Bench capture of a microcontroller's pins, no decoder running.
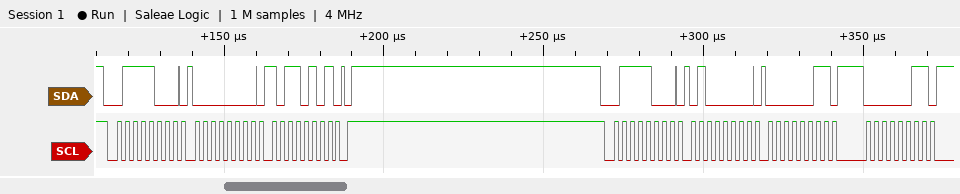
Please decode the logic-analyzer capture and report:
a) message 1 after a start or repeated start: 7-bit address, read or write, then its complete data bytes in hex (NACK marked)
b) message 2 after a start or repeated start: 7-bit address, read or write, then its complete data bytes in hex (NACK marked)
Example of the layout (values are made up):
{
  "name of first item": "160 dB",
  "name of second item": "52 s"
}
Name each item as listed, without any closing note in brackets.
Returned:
{
  "message 1 after a start or repeated start: 7-bit address, read or write, then its complete data bytes in hex": "0x3C write: 00 B5",
  "message 2 after a start or repeated start: 7-bit address, read or write, then its complete data bytes in hex": "0x3C write: 40 03 03"
}
